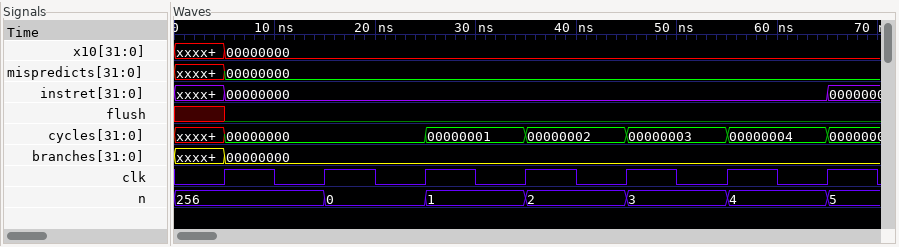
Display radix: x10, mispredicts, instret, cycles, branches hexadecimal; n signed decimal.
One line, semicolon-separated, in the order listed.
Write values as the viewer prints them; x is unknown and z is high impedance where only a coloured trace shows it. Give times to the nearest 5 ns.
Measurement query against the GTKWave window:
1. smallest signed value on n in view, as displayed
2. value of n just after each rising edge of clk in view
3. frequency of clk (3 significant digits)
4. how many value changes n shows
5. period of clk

0; 256, 0, 1, 2, 3, 4, 5; 100 MHz; 6; 10 ns
